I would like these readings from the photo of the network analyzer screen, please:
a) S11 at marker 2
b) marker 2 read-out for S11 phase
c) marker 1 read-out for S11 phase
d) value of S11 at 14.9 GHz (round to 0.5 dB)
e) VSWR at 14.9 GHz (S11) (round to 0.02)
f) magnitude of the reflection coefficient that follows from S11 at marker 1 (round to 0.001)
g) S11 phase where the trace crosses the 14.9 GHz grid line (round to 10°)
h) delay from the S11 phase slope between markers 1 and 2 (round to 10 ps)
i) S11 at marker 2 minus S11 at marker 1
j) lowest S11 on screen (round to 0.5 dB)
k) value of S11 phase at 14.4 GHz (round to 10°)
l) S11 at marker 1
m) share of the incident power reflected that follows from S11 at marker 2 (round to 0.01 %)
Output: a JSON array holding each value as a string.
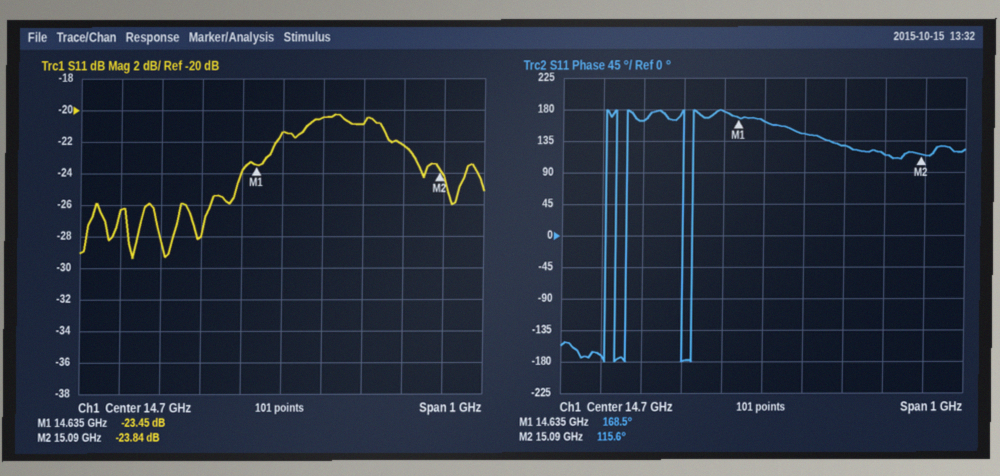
["-23.84 dB", "115.6°", "168.5°", "-21.0 dB", "1.20", "0.067", "130°", "320 ps", "-0.39 dB", "-29.5 dB", "160°", "-23.45 dB", "0.41 %"]
